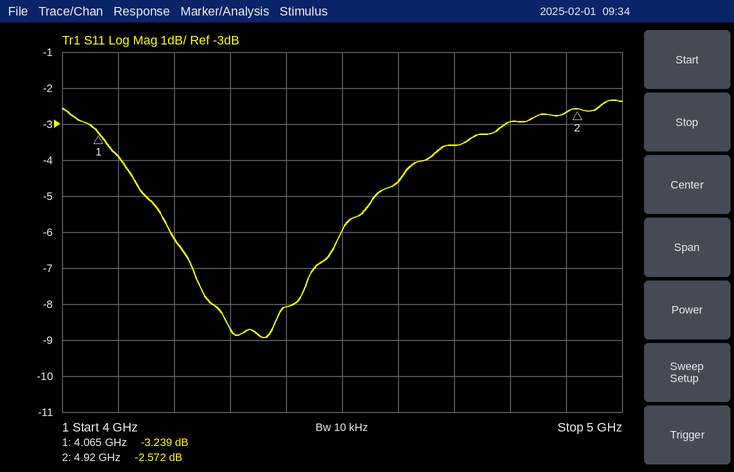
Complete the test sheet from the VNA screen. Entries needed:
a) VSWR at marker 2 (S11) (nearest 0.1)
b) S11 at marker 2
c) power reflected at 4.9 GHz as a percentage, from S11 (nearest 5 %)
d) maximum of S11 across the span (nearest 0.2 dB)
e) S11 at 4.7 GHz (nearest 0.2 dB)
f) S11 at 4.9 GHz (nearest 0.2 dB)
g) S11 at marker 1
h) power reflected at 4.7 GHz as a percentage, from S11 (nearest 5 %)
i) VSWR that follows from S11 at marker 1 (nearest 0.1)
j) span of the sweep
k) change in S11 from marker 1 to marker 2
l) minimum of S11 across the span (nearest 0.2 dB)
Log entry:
6.8
-2.572 dB
55 %
-2.4 dB
-3.6 dB
-2.6 dB
-3.239 dB
45 %
5.4
1 GHz
0.667 dB
-9.0 dB
